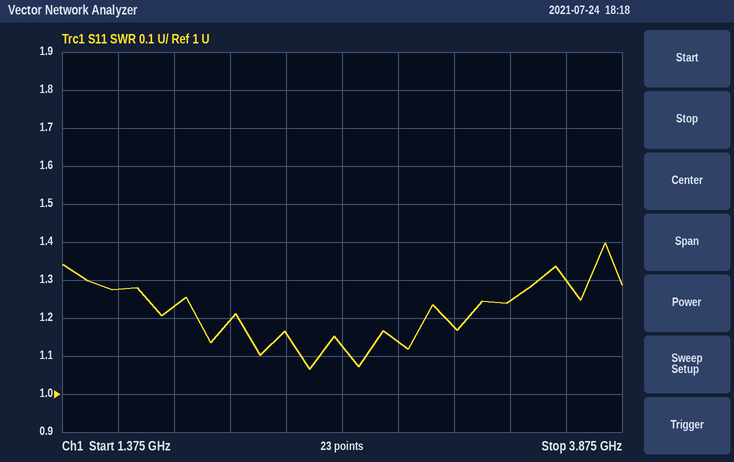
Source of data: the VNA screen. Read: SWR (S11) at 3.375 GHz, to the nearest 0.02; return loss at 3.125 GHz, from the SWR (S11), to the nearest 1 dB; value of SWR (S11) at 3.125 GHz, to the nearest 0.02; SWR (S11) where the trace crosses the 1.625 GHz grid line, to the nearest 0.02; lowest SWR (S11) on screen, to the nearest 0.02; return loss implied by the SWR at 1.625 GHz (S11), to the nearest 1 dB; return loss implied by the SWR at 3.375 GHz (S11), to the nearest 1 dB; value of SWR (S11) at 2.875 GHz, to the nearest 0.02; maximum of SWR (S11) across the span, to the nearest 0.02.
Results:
1.24
22 dB
1.18
1.28
1.06
18 dB
19 dB
1.14
1.40
